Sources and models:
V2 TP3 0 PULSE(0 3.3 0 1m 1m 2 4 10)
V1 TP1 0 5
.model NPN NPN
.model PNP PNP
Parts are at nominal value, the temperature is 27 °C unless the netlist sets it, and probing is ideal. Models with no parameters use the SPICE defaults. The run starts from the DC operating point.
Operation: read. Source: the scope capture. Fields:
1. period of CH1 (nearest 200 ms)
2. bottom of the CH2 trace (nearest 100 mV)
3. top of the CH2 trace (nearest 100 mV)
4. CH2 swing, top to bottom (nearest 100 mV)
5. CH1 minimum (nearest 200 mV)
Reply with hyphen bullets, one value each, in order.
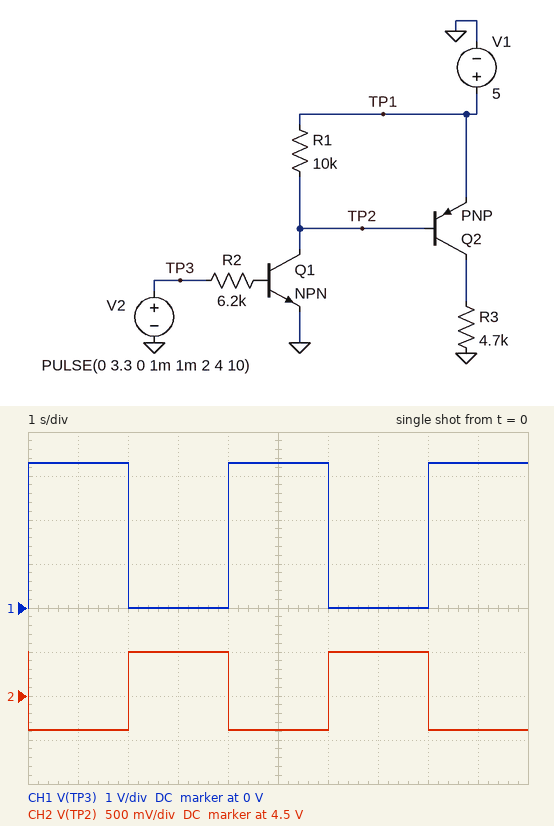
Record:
- 4.0 s
- 4.1 V
- 5.0 V
- 900 mV
- 0 V
